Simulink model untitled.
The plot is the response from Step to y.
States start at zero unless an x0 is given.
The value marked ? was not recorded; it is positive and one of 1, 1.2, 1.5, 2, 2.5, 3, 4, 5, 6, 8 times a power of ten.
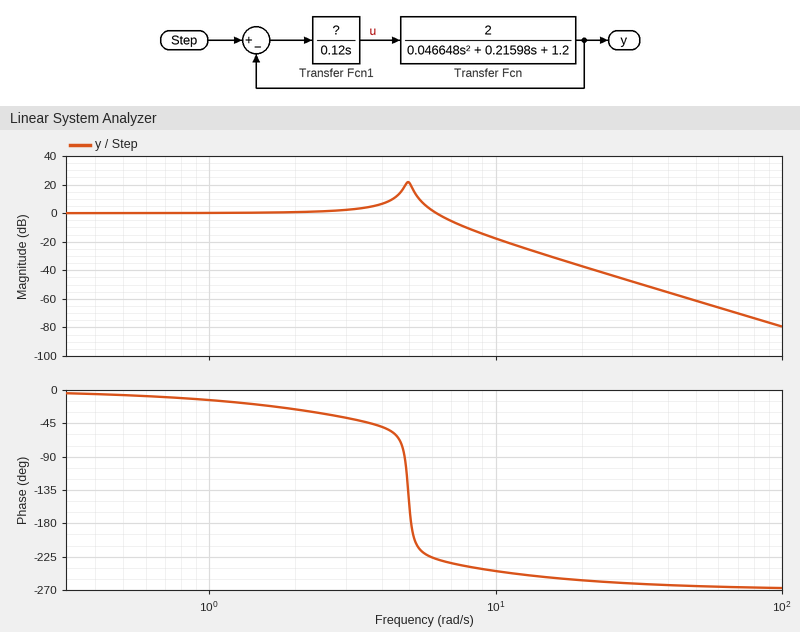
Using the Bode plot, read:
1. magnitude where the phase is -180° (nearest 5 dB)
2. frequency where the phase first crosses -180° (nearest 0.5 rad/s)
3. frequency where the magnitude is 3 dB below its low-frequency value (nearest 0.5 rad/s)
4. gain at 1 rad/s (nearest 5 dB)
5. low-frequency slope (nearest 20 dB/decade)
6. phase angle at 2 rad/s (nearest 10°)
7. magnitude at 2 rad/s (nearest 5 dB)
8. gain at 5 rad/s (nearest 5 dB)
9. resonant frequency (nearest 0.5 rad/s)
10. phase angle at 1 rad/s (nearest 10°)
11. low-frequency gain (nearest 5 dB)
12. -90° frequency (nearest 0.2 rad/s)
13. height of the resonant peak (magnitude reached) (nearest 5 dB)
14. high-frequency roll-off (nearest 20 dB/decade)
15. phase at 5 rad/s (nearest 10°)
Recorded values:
20 dB
5.0 rad/s
6.5 rad/s
0 dB
0 dB/decade
-30°
0 dB
20 dB
5.0 rad/s
-10°
0 dB
4.8 rad/s
20 dB
-60 dB/decade
-160°
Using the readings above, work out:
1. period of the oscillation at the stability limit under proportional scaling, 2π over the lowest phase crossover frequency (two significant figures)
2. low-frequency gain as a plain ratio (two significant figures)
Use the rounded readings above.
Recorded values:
1.3 s
1.0
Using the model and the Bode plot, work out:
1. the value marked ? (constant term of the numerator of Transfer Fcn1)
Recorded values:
0.3
